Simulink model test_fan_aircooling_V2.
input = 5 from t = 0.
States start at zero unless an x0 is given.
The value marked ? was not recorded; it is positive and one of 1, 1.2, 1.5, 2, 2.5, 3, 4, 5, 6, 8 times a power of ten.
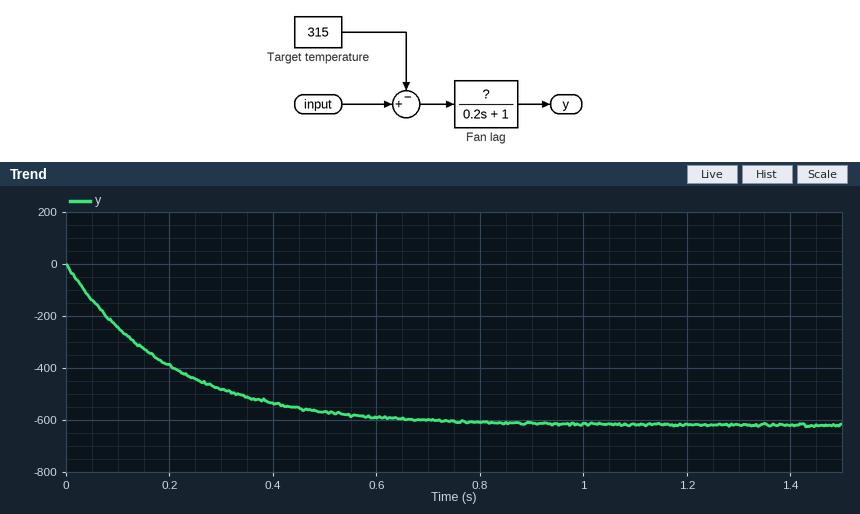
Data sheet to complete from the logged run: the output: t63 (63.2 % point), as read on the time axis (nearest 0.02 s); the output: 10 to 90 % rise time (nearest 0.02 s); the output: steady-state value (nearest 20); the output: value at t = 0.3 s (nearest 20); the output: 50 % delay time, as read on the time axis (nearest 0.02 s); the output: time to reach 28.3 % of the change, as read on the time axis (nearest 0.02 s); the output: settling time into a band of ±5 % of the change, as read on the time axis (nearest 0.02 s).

0.20 s
0.44 s
-620
-480
0.14 s
0.06 s
0.60 s
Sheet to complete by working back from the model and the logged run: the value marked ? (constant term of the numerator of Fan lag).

2
